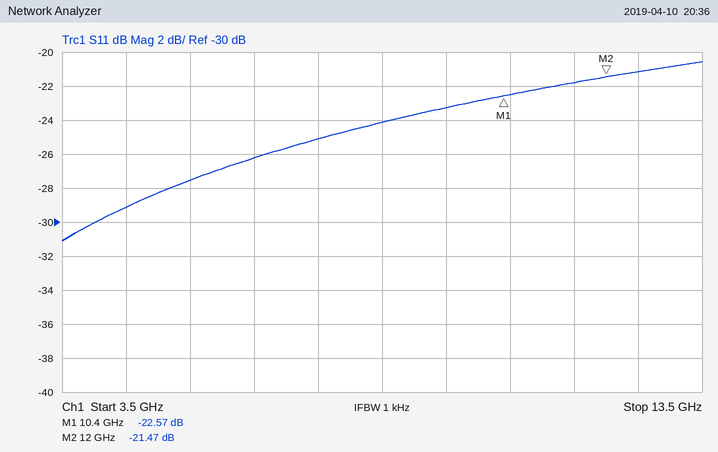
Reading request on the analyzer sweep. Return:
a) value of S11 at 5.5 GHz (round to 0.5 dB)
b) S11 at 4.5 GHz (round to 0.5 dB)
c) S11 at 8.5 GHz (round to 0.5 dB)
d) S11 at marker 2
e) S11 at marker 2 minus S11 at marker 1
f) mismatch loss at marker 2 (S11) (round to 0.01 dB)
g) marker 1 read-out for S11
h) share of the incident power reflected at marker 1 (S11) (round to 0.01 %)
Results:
-27.5 dB
-29.0 dB
-24.0 dB
-21.47 dB
1.10 dB
0.03 dB
-22.57 dB
0.55 %
